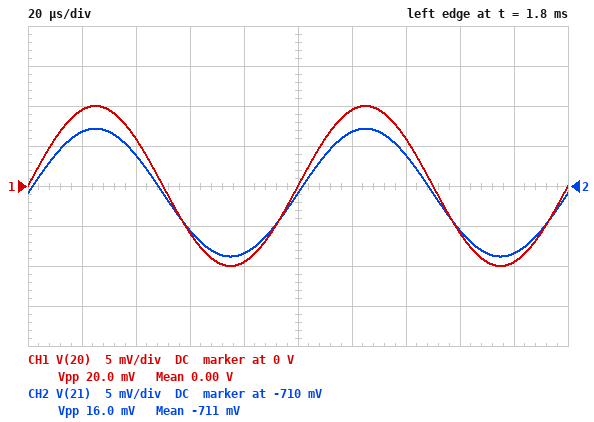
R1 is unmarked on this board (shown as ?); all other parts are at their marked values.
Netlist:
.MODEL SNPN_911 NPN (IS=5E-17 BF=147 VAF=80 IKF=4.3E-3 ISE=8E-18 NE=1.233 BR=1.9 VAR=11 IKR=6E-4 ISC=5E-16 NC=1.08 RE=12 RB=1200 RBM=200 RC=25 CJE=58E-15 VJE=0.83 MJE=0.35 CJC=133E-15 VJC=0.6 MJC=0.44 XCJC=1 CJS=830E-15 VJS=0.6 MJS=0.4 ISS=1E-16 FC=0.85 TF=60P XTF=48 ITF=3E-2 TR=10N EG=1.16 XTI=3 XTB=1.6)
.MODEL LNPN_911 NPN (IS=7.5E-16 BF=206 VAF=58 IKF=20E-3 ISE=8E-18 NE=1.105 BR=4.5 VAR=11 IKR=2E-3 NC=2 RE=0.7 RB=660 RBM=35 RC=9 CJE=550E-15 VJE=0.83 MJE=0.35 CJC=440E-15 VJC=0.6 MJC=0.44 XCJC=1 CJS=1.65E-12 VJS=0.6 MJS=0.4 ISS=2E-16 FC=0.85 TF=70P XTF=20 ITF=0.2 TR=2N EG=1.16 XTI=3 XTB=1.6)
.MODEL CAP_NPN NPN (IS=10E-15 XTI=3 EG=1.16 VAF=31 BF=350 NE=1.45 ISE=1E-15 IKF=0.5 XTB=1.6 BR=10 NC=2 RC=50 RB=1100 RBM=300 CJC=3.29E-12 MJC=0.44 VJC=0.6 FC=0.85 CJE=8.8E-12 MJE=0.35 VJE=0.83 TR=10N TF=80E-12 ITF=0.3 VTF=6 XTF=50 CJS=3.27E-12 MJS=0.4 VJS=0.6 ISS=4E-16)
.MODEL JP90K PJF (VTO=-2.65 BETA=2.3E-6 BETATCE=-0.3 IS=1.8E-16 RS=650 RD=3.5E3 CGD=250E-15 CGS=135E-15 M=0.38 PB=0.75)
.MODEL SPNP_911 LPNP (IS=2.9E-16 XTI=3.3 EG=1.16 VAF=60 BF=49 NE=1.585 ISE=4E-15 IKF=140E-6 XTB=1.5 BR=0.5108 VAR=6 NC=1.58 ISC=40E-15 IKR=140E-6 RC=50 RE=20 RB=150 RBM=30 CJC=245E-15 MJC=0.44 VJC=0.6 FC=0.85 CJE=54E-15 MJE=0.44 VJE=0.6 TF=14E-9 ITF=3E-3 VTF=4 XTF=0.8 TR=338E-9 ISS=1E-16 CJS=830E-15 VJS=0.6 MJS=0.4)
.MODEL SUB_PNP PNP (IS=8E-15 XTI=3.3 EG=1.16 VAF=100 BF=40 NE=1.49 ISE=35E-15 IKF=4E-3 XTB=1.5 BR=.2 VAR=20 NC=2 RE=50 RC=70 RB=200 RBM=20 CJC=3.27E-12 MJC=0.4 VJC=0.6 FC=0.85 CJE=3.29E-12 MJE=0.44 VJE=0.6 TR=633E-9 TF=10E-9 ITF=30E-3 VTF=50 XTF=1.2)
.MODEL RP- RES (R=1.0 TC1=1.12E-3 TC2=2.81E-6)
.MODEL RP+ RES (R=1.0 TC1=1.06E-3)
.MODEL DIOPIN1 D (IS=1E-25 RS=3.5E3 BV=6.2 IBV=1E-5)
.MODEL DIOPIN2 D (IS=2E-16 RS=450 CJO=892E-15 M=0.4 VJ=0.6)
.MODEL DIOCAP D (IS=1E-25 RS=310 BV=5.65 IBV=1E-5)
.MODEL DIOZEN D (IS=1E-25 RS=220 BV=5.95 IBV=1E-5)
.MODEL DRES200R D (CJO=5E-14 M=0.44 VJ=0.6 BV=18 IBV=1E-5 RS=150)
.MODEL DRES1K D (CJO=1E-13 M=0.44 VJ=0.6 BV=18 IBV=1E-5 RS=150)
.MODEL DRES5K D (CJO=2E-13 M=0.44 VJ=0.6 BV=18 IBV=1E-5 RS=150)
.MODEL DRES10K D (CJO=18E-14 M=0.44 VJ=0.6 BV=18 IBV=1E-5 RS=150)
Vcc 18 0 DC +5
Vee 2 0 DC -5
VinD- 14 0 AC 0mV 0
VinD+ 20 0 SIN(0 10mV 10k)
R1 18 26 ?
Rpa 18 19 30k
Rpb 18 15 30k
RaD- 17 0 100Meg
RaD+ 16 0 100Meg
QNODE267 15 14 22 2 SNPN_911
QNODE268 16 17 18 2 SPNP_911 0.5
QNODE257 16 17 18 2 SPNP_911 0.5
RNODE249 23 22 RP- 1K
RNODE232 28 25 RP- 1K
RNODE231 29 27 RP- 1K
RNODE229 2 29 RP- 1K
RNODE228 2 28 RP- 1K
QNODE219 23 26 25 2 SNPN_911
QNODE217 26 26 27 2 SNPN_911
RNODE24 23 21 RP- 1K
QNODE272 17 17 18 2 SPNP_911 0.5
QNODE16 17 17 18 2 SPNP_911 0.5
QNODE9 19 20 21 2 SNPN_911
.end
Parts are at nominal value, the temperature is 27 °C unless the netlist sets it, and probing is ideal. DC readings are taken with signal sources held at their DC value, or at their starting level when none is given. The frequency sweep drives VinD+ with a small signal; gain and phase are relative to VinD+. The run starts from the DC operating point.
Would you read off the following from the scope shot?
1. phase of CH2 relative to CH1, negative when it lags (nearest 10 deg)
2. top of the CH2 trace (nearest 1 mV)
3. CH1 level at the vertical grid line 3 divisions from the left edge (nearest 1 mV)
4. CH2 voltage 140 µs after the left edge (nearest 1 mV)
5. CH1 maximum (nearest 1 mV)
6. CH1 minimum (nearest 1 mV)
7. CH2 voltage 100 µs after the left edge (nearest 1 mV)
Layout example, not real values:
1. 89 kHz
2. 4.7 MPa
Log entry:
1. 0 deg
2. -703 mV
3. -6 mV
4. -706 mV
5. 10 mV
6. -10 mV
7. -711 mV
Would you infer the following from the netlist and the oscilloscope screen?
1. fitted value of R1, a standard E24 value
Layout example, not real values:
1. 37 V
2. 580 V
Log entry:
1. 110 kΩ
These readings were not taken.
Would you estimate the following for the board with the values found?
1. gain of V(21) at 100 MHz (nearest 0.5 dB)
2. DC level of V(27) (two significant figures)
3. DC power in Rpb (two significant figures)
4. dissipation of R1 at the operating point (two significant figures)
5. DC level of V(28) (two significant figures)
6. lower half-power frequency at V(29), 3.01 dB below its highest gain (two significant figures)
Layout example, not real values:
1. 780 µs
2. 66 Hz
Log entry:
1. -2.5 dB
2. -4.8 V
3. 50 µW
4. 750 µW
5. -4.9 V
6. 67 MHz
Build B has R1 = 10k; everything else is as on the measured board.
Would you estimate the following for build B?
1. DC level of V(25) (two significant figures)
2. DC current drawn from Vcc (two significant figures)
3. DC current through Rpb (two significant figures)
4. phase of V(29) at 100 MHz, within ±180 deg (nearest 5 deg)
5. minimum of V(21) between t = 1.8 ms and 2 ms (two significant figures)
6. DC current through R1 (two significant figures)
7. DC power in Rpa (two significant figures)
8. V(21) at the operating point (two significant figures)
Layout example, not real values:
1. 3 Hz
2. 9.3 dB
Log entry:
1. -3.5 V
2. 1.2 mA
3. 200 µA
4. 25 deg
5. -960 mV
6. 770 µA
7. 1.2 mW
8. -950 mV
